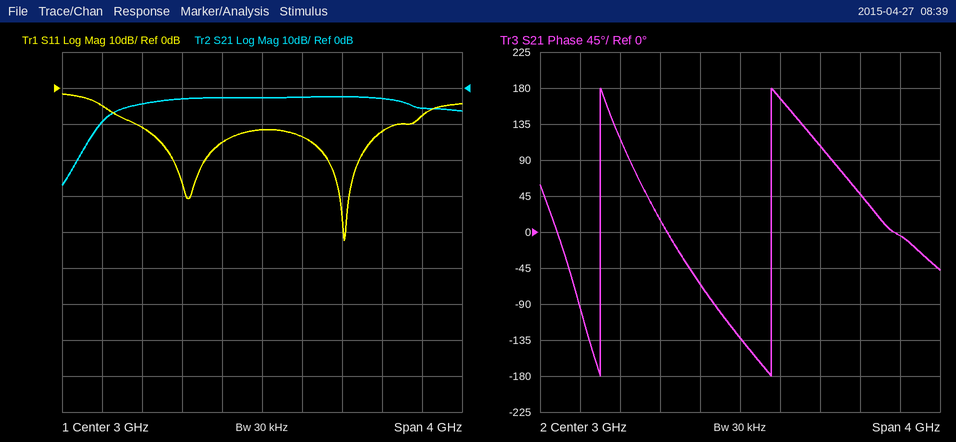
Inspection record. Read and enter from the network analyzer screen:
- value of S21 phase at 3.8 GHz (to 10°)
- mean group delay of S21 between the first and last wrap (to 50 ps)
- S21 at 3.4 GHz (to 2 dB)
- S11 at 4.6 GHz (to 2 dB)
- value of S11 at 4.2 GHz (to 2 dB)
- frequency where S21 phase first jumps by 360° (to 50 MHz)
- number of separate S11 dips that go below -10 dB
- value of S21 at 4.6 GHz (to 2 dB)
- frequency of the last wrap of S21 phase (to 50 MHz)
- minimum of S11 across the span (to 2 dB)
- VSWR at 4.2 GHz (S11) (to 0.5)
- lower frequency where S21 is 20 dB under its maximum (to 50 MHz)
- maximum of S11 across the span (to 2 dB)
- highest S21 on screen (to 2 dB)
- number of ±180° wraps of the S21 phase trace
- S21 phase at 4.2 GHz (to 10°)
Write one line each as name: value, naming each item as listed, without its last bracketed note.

value of S21 phase at 3.8 GHz: 110°
mean group delay of S21 between the first and last wrap: 600 ps
S21 at 3.4 GHz: -2 dB
S11 at 4.6 GHz: -8 dB
value of S11 at 4.2 GHz: -12 dB
frequency where S21 phase first jumps by 360°: 1.60 GHz
number of separate S11 dips that go below -10 dB: 2
value of S21 at 4.6 GHz: -6 dB
frequency of the last wrap of S21 phase: 3.30 GHz
minimum of S11 across the span: -42 dB
VSWR at 4.2 GHz (S11): 1.5
lower frequency where S21 is 20 dB under its maximum: 1.10 GHz
maximum of S11 across the span: -2 dB
highest S21 on screen: -2 dB
number of ±180° wraps of the S21 phase trace: 2
S21 phase at 4.2 GHz: 50°
